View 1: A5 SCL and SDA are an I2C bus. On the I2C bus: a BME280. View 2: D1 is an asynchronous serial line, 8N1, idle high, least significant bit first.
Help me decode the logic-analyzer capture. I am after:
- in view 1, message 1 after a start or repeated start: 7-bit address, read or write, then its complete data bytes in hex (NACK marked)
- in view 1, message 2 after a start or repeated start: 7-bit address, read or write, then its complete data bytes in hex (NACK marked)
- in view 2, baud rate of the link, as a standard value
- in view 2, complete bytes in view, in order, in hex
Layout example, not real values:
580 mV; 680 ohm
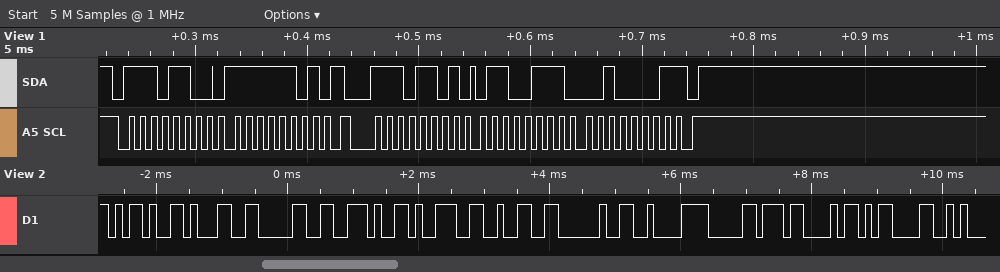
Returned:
0x76 write: FD; 0x76 read: 67 21 NACK; 9600 baud; 2D 31 30 2E 39 32 20 C2 B0 43 0D
